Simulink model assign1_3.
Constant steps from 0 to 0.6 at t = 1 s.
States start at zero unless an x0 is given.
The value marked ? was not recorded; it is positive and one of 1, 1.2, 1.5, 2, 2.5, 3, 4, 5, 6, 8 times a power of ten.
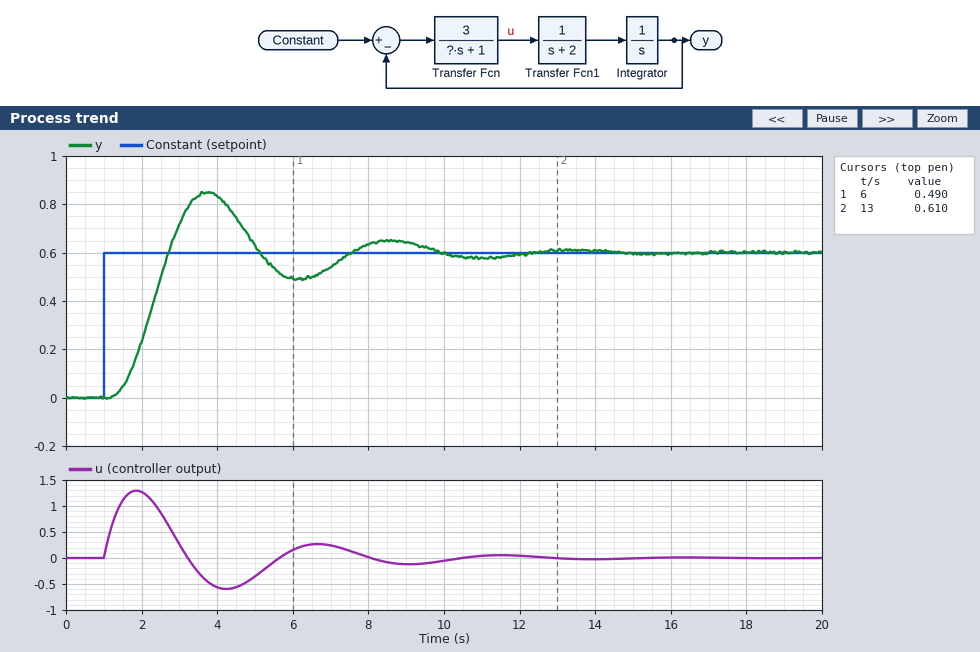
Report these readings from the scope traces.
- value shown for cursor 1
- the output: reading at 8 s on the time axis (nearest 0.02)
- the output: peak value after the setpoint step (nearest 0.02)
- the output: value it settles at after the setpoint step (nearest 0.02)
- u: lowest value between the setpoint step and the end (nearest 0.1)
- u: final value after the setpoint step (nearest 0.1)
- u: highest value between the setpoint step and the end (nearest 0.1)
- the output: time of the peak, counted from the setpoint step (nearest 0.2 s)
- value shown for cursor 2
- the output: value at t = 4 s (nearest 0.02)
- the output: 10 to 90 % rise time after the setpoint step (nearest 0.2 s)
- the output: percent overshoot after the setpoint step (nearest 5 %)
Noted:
0.490
0.64
0.84
0.60
-0.6
0.0
1.3
2.8 s
0.610
0.84
1.0 s
40 %
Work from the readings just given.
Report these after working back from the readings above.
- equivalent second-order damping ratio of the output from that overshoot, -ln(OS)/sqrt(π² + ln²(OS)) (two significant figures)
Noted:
0.28
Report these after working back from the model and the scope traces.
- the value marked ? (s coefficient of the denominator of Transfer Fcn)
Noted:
0.5
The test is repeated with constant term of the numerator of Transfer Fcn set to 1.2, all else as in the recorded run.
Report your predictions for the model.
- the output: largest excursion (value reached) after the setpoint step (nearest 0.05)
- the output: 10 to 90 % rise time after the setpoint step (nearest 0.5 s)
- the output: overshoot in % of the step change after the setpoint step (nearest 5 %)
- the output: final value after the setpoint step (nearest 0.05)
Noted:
0.65
2.0 s
10 %
0.60
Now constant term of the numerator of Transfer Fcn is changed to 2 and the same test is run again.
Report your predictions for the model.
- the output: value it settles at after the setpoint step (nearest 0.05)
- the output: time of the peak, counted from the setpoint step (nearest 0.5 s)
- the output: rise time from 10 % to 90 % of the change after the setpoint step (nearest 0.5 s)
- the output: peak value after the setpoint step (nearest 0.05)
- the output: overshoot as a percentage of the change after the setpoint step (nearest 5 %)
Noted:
0.60
3.5 s
1.5 s
0.75
25 %
